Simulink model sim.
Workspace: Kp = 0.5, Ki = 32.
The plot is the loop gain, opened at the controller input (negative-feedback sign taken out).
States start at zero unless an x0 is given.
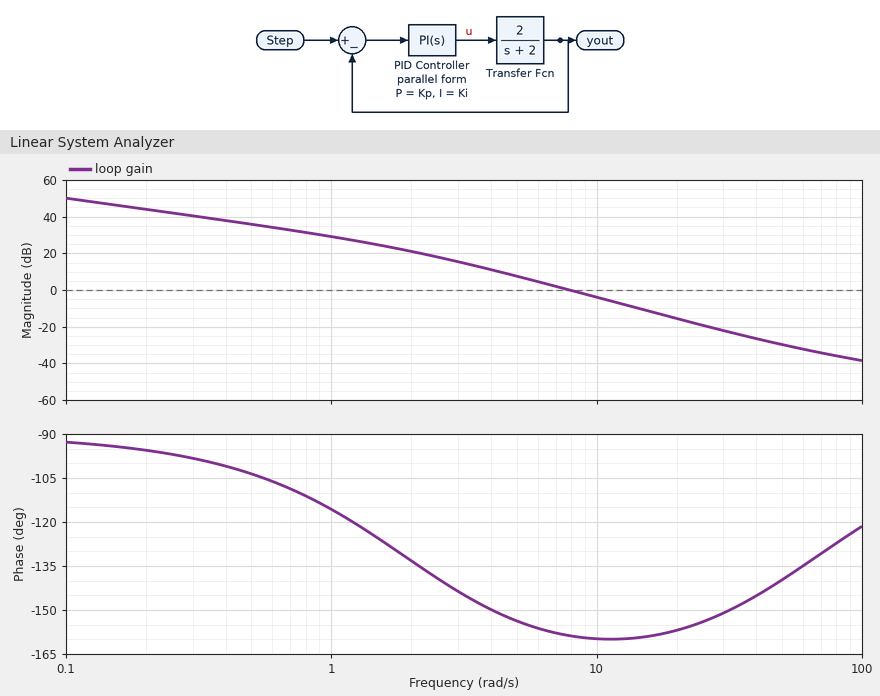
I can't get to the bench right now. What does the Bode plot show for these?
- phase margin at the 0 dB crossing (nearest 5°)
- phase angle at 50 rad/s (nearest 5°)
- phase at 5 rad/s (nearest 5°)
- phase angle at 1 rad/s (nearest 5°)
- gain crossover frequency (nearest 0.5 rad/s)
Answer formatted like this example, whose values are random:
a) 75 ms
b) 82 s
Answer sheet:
a) 20°
b) -140°
c) -155°
d) -115°
e) 8.0 rad/s
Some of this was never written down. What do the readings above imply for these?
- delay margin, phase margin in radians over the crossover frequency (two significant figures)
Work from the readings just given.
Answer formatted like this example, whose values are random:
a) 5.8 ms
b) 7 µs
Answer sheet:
a) 0.044 s
